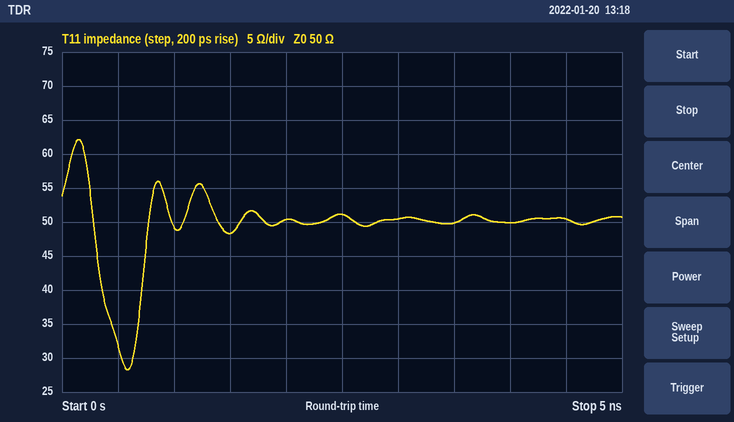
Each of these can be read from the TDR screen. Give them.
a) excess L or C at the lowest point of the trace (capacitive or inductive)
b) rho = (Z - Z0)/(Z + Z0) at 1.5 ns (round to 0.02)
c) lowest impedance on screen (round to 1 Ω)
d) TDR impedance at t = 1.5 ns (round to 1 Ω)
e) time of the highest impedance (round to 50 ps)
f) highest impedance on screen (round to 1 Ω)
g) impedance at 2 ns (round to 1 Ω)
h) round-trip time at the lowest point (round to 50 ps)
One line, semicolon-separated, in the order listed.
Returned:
capacitive; -0.02; 28 Ω; 48 Ω; 150 ps; 62 Ω; 50 Ω; 600 ps
